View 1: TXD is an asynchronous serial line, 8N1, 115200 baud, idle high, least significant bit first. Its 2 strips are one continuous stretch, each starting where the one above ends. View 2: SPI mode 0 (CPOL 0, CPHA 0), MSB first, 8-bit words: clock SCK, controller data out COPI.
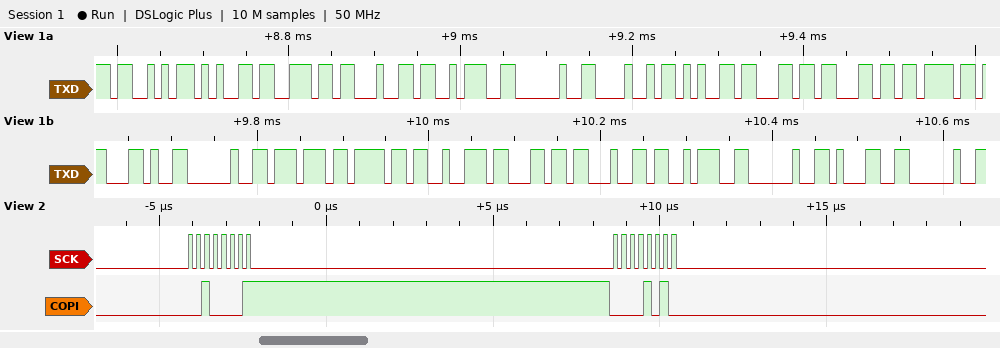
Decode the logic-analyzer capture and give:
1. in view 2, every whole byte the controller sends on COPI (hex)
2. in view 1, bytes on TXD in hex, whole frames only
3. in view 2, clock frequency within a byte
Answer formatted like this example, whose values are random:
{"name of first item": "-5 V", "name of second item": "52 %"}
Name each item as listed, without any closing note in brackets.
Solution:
{"in view 2, every whole byte the controller sends on COPI": "21 0A", "in view 1, bytes on TXD in hex, whole frames only": "53 65 6E 64 3A 20 48 65 6C 6C 6F 2C 20 77 6F 72 6C 64 3A 20 31 20", "in view 2, clock frequency within a byte": "4 MHz"}
